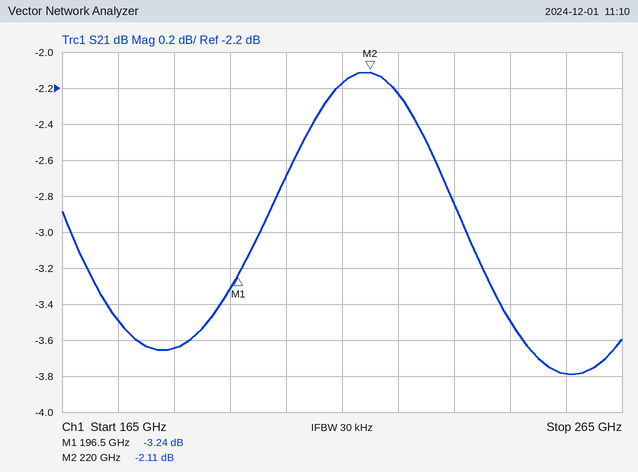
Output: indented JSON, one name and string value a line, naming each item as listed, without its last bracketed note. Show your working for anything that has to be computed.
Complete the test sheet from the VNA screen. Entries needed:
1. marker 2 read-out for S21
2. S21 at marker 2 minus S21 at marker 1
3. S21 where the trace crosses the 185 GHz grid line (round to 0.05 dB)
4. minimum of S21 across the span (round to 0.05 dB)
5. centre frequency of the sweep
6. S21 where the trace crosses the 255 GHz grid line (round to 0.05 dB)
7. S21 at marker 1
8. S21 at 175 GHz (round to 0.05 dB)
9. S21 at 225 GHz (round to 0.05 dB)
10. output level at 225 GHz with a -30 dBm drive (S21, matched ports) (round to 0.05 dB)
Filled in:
{
  "marker 2 read-out for S21": "-2.11 dB",
  "S21 at marker 2 minus S21 at marker 1": "-2.11 − (-3.24) = 1.13 dB",
  "S21 where the trace crosses the 185 GHz grid line": "-3.65 dB",
  "minimum of S21 across the span": "-3.80 dB",
  "centre frequency of the sweep": "215 GHz",
  "S21 where the trace crosses the 255 GHz grid line": "-3.80 dB",
  "S21 at marker 1": "-3.24 dB",
  "S21 at 175 GHz": "-3.50 dB",
  "S21 at 225 GHz": "-2.25 dB",
  "output level at 225 GHz with a -30 dBm drive (S21, matched ports)": "-30 dBm + (-2.25 dB) = -32.25 dBm"
}
